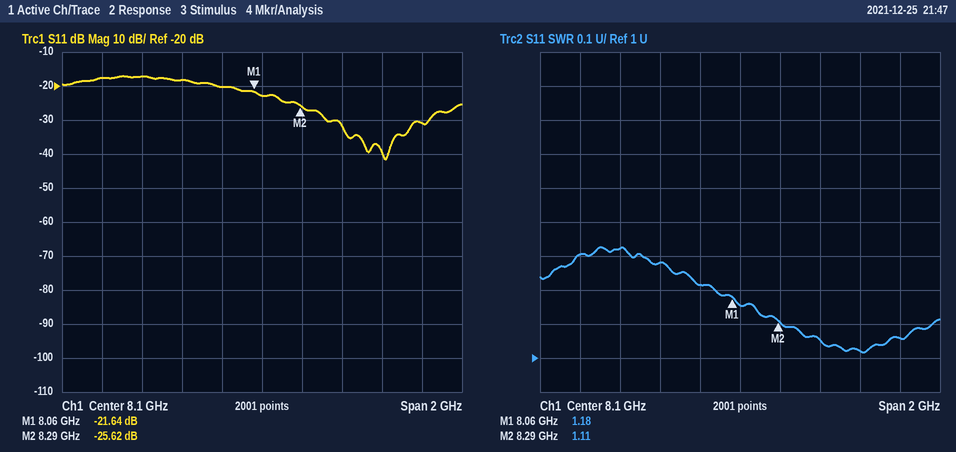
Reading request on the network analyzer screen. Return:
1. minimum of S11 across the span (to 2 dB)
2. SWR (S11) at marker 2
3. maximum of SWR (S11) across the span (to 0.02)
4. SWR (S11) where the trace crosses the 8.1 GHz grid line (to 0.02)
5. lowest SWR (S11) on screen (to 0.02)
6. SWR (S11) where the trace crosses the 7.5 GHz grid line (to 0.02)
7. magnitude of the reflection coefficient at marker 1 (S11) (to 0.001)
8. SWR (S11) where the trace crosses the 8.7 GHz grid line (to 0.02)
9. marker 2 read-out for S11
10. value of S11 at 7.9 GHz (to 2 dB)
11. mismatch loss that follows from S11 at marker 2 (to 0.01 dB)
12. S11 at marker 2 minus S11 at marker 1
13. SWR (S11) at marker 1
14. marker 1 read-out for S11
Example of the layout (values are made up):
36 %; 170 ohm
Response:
-42 dB; 1.11; 1.32; 1.16; 1.02; 1.32; 0.083; 1.02; -25.62 dB; -20 dB; 0.01 dB; -3.98 dB; 1.18; -21.64 dB
